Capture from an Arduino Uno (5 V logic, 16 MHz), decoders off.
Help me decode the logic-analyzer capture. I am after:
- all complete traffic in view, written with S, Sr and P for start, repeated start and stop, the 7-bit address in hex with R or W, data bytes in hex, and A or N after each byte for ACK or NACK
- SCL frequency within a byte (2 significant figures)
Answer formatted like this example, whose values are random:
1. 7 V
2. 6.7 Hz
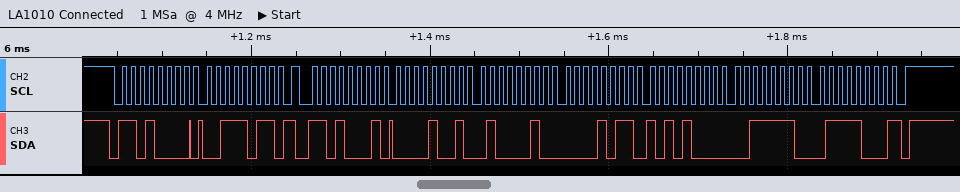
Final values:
1. S 68W A 3B A Sr 68R A 09 A 42 A 0B A A8 A 3E A 78 N P
2. 100 kHz
